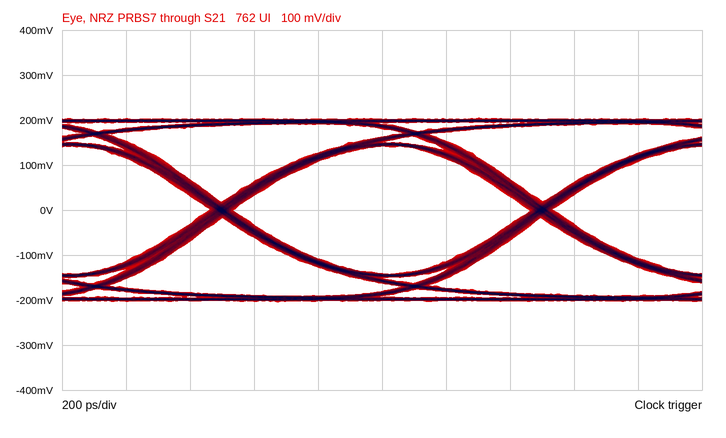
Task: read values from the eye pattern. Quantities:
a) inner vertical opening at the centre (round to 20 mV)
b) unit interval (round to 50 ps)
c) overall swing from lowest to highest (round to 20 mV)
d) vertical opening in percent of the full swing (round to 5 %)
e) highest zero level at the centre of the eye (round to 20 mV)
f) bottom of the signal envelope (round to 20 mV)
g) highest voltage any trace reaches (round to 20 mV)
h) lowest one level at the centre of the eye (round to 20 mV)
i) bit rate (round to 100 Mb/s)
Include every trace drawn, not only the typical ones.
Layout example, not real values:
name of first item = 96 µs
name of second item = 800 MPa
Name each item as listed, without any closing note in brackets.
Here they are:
inner vertical opening at the centre = 280 mV
unit interval = 1.00 ns
overall swing from lowest to highest = 400 mV
vertical opening in percent of the full swing = 70 %
highest zero level at the centre of the eye = -140 mV
bottom of the signal envelope = -200 mV
highest voltage any trace reaches = 200 mV
lowest one level at the centre of the eye = 140 mV
bit rate = 1.0 Gb/s
